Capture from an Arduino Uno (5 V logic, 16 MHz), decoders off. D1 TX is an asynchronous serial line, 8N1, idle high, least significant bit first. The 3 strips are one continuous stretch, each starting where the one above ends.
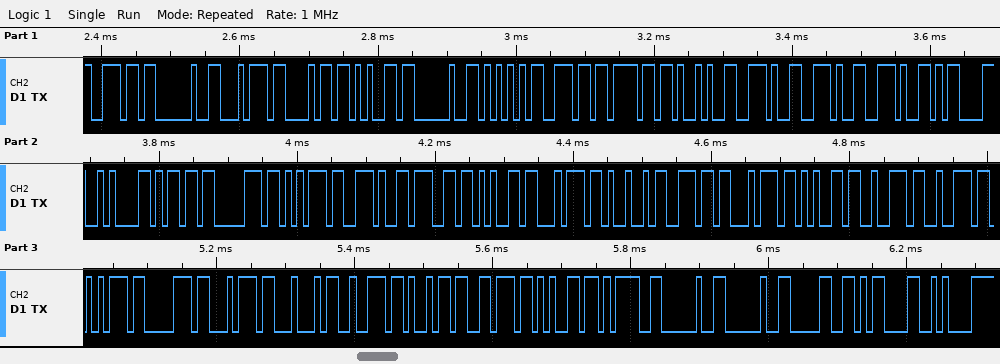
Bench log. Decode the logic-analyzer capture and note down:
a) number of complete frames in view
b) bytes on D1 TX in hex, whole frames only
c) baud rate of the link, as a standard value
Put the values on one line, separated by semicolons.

42; 6E 20 74 68 65 20 55 6E 6F 29 2E 2E 2E 0D 0A 6D 70 75 2E 67 65 74 49 6E 74 65 72 72 75 70 74 44 72 69 76 65 3D 20 20 30 0D 0A; 115200 baud
